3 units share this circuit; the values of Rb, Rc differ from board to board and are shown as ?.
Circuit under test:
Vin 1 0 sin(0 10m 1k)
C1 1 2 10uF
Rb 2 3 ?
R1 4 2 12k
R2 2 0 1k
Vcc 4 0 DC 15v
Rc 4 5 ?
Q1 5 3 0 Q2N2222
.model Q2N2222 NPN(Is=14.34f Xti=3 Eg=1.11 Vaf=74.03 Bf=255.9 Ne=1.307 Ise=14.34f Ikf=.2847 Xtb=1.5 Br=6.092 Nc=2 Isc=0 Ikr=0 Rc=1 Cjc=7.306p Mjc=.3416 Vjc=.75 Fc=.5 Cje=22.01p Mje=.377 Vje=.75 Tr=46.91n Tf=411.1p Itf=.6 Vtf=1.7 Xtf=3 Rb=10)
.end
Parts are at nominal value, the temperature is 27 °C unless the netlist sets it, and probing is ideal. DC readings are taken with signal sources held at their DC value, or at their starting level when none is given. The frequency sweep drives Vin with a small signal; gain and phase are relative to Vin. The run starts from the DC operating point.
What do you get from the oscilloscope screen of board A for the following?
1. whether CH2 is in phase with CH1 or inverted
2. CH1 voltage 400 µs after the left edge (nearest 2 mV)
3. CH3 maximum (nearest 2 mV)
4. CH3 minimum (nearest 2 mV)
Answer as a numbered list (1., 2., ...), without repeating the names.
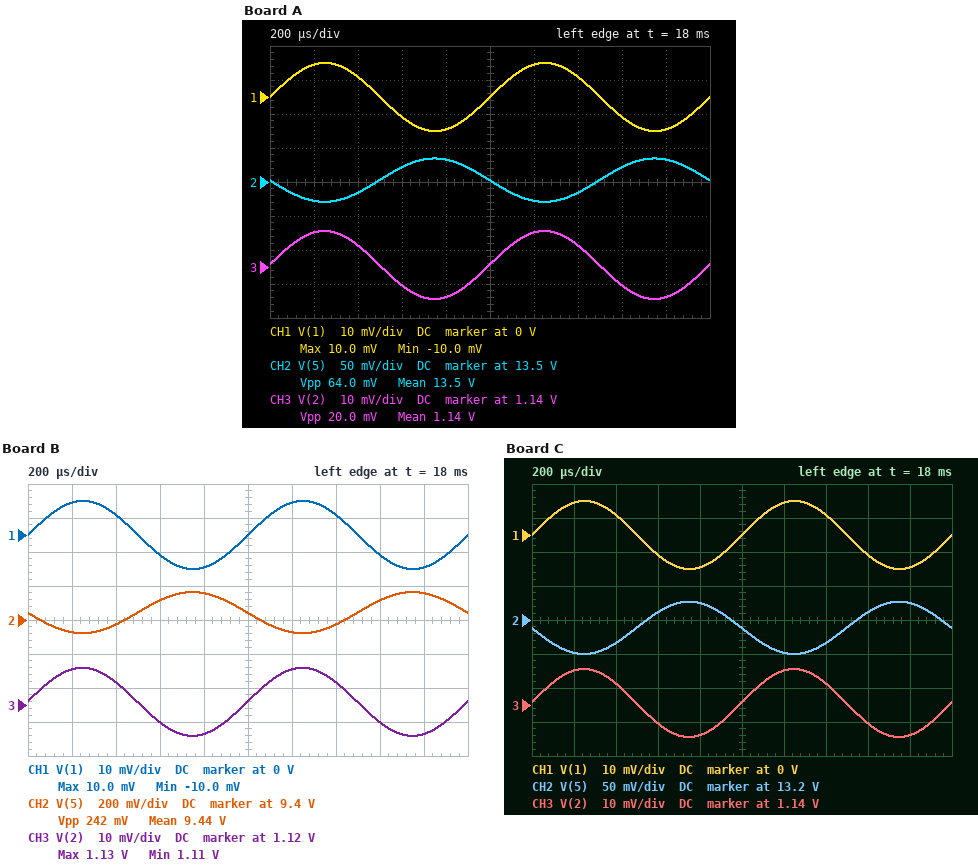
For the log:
1. inverted
2. 6 mV
3. 1.150 V
4. 1.130 V
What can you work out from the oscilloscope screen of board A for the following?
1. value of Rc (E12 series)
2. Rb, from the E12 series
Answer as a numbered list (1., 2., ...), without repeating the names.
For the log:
1. 560 Ω
2. 33 kΩ
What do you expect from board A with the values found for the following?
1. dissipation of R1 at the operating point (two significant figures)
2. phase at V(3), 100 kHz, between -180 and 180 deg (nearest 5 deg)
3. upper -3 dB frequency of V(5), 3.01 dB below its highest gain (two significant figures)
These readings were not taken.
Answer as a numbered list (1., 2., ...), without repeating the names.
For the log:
1. 16 mW
2. -15 deg
3. 360 kHz
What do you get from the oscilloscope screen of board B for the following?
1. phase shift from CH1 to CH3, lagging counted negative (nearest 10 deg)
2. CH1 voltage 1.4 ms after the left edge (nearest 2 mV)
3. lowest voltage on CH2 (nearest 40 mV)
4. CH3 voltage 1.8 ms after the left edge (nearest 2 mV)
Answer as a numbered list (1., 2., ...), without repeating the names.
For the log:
1. 0 deg
2. 6 mV
3. 9.32 V
4. 1.112 V
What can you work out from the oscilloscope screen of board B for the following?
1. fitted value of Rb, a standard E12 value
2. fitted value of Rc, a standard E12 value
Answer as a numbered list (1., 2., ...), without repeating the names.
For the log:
1. 12 kΩ
2. 820 Ω
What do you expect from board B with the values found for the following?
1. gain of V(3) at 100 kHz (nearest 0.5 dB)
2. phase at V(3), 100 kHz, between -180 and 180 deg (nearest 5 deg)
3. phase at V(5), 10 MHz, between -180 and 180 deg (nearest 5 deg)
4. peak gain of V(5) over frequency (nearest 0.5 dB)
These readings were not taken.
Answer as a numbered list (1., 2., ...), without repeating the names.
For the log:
1. -24.5 dB
2. -20 deg
3. 90 deg
4. 21.5 dB
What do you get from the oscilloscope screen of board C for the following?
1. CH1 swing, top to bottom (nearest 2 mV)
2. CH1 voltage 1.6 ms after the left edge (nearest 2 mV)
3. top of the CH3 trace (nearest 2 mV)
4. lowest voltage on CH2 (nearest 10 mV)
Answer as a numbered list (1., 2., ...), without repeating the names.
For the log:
1. 20 mV
2. -6 mV
3. 1.150 V
4. 13.15 V
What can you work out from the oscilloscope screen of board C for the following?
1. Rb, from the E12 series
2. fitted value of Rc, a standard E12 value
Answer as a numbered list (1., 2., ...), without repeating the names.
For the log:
1. 33 kΩ
2. 680 Ω
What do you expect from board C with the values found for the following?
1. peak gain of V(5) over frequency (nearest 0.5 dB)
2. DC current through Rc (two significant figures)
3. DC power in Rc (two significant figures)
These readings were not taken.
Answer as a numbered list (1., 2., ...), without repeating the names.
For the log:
1. 11.5 dB
2. 2.7 mA
3. 4.8 mW
